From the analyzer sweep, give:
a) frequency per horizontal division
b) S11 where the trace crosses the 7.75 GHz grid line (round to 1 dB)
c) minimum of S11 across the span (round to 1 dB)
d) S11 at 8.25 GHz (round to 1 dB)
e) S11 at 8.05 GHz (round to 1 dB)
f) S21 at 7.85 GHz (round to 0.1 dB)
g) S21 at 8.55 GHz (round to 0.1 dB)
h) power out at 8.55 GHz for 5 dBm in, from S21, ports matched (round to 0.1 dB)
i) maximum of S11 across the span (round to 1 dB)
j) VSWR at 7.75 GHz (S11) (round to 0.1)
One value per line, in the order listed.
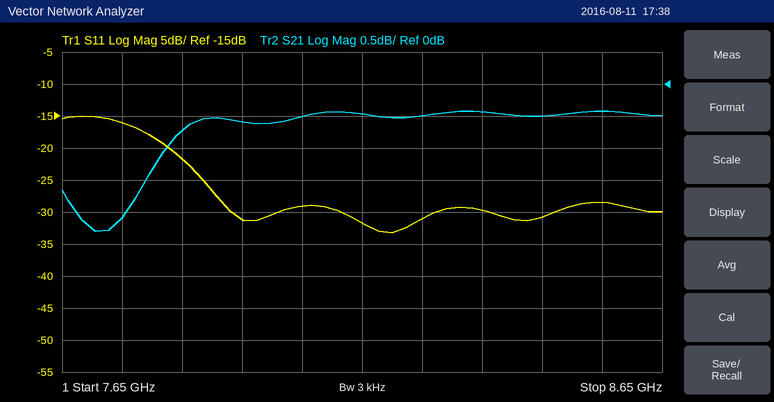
100 MHz
-16 dB
-33 dB
-31 dB
-29 dB
-0.7 dB
-0.4 dB
4.6 dBm
-15 dB
1.4
